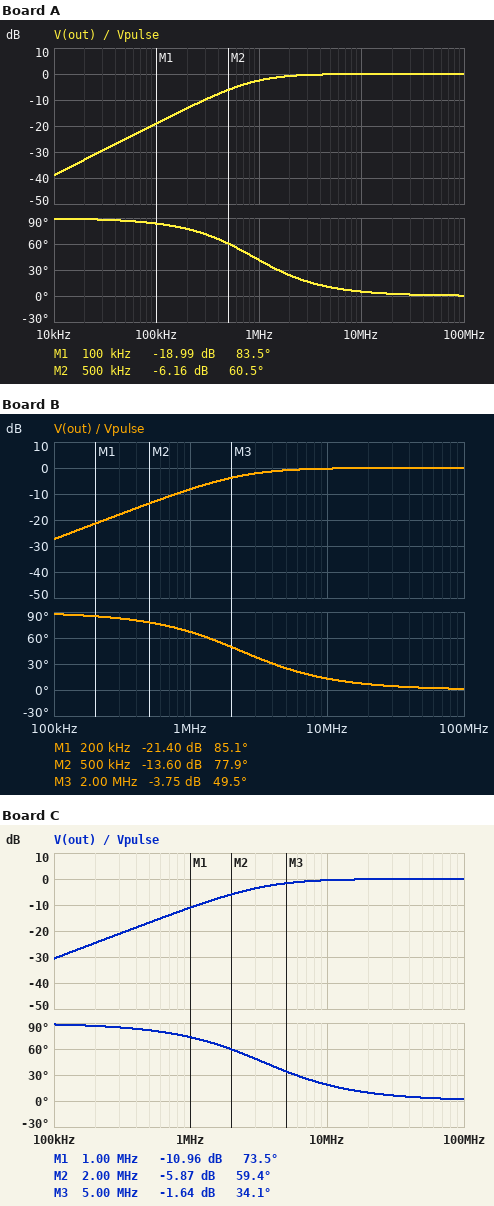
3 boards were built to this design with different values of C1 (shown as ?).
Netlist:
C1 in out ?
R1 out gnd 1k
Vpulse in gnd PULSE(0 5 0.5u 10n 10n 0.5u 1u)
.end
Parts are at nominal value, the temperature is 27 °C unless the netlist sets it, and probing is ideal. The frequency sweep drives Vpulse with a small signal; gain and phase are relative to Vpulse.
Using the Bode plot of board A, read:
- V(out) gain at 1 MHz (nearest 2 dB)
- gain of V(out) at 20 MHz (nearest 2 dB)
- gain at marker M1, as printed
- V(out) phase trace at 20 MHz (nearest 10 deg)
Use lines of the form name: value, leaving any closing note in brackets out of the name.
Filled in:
V(out) gain at 1 MHz: -2 dB
gain of V(out) at 20 MHz: 0 dB
gain at marker M1, as printed: -18.99 dB
V(out) phase trace at 20 MHz: 0 deg
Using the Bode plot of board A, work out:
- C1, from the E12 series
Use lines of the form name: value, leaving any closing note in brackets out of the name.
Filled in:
C1, from the E12 series: 180 pF
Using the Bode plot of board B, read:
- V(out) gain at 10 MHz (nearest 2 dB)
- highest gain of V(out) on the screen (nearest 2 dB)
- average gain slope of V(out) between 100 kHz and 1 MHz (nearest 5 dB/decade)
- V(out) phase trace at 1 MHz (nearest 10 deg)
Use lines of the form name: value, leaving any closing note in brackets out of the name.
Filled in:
V(out) gain at 10 MHz: 0 dB
highest gain of V(out) on the screen: 0 dB
average gain slope of V(out) between 100 kHz and 1 MHz: 20 dB/decade
V(out) phase trace at 1 MHz: 70 deg
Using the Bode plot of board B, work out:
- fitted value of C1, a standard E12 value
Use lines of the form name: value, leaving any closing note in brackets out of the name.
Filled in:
fitted value of C1, a standard E12 value: 68 pF
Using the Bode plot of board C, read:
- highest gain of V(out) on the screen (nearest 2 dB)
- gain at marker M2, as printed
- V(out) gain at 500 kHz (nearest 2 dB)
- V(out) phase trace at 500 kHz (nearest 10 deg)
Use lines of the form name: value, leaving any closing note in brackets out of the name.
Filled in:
highest gain of V(out) on the screen: 0 dB
gain at marker M2, as printed: -5.87 dB
V(out) gain at 500 kHz: -16 dB
V(out) phase trace at 500 kHz: 80 deg
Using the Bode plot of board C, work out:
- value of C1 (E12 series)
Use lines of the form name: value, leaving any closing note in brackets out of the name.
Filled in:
value of C1: 47 pF
